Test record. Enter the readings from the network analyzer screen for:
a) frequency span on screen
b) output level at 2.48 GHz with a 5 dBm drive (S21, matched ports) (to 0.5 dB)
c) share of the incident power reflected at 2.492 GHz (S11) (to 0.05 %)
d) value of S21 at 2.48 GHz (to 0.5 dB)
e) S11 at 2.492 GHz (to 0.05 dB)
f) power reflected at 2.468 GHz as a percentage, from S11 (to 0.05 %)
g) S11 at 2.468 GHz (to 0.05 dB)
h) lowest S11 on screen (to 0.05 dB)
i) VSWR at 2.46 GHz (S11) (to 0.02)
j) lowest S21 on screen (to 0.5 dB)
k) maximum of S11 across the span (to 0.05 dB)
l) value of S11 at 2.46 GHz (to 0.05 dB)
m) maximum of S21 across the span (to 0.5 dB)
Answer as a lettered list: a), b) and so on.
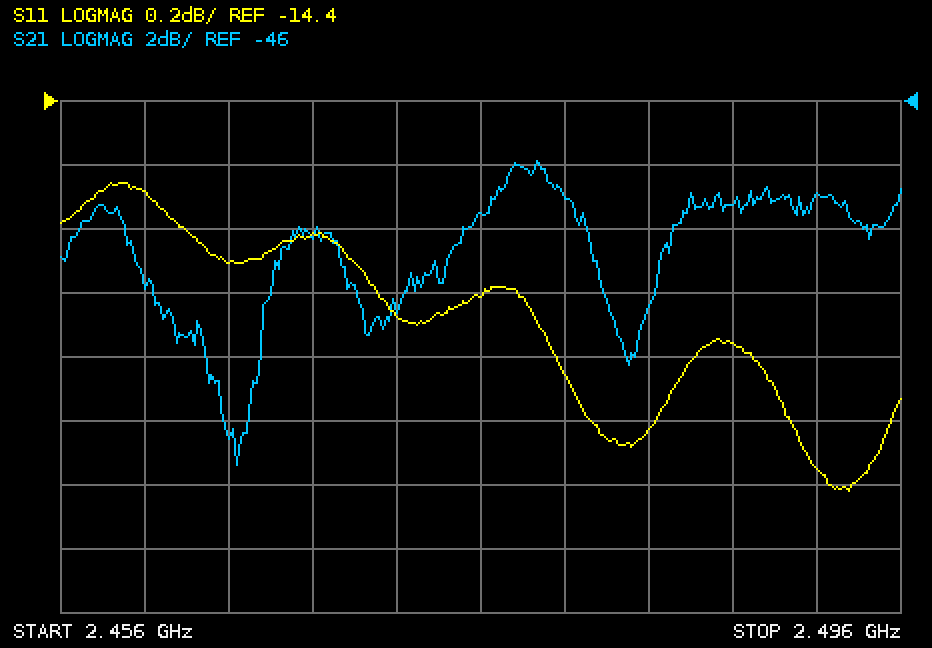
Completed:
a) 40 MHz
b) -44.0 dBm
c) 2.80 %
d) -49.0 dB
e) -15.55 dB
f) 3.30 %
g) -14.80 dB
h) -15.60 dB
i) 1.46
j) -57.5 dB
k) -14.65 dB
l) -14.70 dB
m) -48.0 dB
